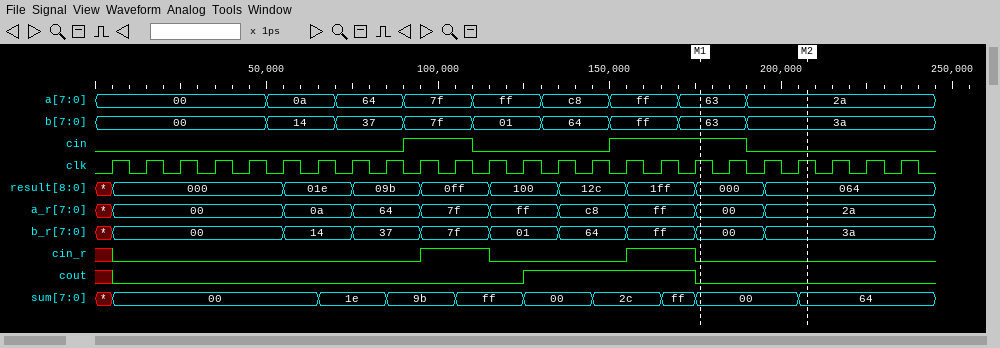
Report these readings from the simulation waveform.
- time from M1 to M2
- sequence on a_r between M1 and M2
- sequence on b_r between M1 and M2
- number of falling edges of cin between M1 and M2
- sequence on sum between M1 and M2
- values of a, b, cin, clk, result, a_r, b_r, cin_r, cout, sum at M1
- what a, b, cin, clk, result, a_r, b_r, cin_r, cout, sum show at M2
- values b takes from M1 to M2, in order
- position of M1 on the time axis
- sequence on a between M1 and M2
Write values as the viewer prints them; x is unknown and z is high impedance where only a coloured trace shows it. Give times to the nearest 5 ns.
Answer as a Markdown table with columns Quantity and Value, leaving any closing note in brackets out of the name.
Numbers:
| Quantity | Value |
|---|---|
| time from M1 to M2 | 30 ns |
| sequence on a_r between M1 and M2 | 00, 2a |
| sequence on b_r between M1 and M2 | 00, 3a |
| number of falling edges of cin between M1 and M2 | 1 |
| sequence on sum between M1 and M2 | 00, 64 |
| values of a, b, cin, clk, result, a_r, b_r, cin_r, cout, sum at M1 | a=63, b=63, cin=1, clk=1, result=000, a_r=00, b_r=00, cin_r=0, cout=0, sum=00 |
| what a, b, cin, clk, result, a_r, b_r, cin_r, cout, sum show at M2 | a=2a, b=3a, cin=0, clk=1, result=064, a_r=2a, b_r=3a, cin_r=0, cout=0, sum=64 |
| values b takes from M1 to M2, in order | 63, 3a |
| position of M1 on the time axis | 175 ns |
| sequence on a between M1 and M2 | 63, 2a |
